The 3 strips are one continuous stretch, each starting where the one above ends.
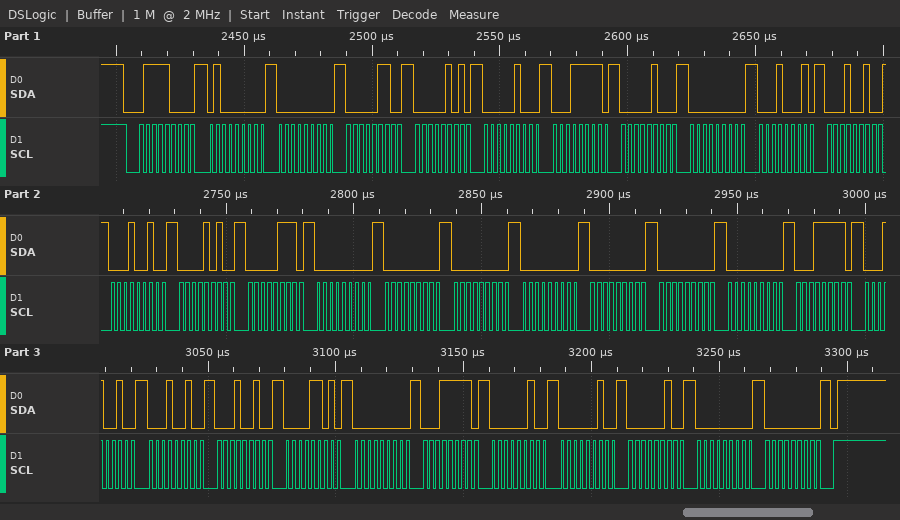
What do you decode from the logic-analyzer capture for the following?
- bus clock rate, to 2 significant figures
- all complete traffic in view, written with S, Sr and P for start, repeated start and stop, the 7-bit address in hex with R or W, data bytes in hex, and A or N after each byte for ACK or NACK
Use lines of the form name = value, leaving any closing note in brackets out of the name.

bus clock rate, to 2 significant figures = 400 kHz
all complete traffic in view, written with S, Sr and P for start, repeated start and stop, the 7-bit address in hex with R or W, data bytes in hex, and A or N after each byte for ACK or NACK = S 3CW A 40 A 00 A 06 A 05 A 04 A 1F A 04 A 00 A 11 A 12 A 12 A 0A A 07 A 00 A 00 A 00 A 00 A 00 A 00 A 00 A 1F A 12 A 12 A 12 A 0D A 00 A 1F A 02 A 02 A 02 A 00 A 00 A P
